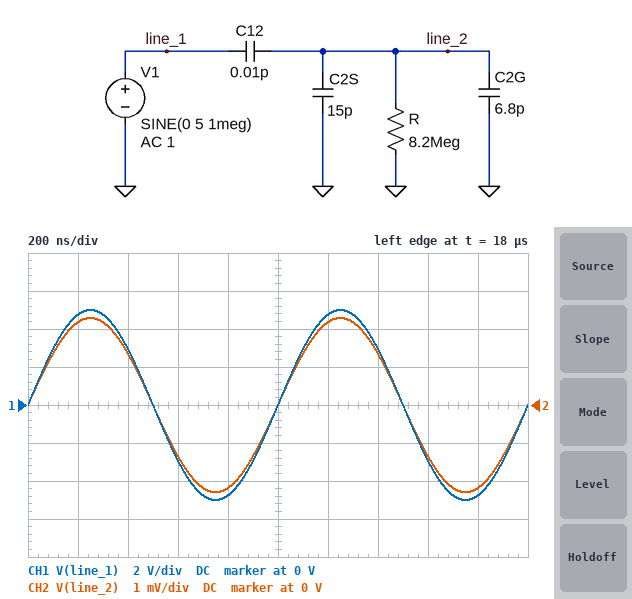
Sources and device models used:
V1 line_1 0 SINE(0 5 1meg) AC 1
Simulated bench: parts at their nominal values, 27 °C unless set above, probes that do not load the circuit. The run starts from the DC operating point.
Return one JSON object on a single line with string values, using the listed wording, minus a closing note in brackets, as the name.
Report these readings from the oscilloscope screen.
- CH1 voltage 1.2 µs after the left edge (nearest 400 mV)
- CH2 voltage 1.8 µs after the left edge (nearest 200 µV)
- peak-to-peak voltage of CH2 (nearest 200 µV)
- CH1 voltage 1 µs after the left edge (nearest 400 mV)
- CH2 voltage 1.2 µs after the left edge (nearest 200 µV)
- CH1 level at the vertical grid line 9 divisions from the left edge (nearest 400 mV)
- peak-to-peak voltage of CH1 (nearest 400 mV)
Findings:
{"CH1 voltage 1.2 µs after the left edge": "4.8 V", "CH2 voltage 1.8 µs after the left edge": "-2.2 mV", "peak-to-peak voltage of CH2": "4.6 mV", "CH1 voltage 1 µs after the left edge": "0 V", "CH2 voltage 1.2 µs after the left edge": "2.2 mV", "CH1 level at the vertical grid line 9 divisions from the left edge": "-4.8 V", "peak-to-peak voltage of CH1": "10.0 V"}
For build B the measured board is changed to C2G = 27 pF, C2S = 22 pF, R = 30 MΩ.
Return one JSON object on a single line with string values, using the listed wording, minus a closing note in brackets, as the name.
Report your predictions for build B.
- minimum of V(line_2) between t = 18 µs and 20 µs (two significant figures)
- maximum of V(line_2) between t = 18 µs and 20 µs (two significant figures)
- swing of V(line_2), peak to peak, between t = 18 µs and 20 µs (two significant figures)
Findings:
{"minimum of V(line_2) between t = 18 µs and 20 µs": "-1.0 mV", "maximum of V(line_2) between t = 18 µs and 20 µs": "1.0 mV", "swing of V(line_2), peak to peak, between t = 18 µs and 20 µs": "2.0 mV"}
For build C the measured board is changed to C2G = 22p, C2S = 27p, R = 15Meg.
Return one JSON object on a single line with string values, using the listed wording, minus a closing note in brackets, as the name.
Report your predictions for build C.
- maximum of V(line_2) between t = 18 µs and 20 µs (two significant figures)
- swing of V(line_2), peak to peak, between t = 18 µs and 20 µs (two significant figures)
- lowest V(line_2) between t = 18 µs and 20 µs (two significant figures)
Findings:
{"maximum of V(line_2) between t = 18 µs and 20 µs": "1.0 mV", "swing of V(line_2), peak to peak, between t = 18 µs and 20 µs": "2.0 mV", "lowest V(line_2) between t = 18 µs and 20 µs": "-1.0 mV"}
